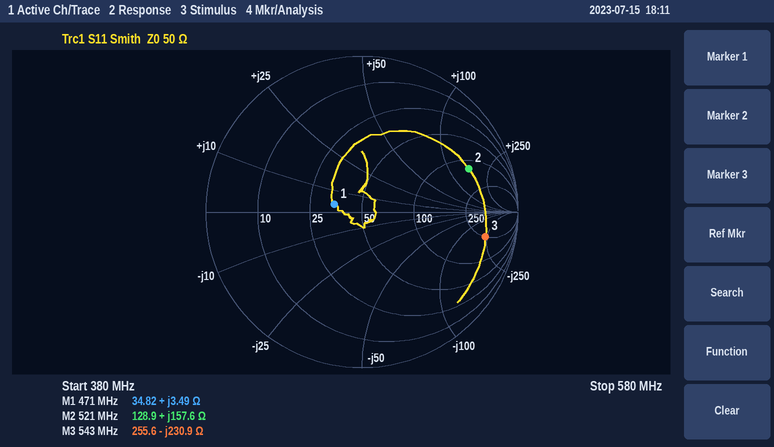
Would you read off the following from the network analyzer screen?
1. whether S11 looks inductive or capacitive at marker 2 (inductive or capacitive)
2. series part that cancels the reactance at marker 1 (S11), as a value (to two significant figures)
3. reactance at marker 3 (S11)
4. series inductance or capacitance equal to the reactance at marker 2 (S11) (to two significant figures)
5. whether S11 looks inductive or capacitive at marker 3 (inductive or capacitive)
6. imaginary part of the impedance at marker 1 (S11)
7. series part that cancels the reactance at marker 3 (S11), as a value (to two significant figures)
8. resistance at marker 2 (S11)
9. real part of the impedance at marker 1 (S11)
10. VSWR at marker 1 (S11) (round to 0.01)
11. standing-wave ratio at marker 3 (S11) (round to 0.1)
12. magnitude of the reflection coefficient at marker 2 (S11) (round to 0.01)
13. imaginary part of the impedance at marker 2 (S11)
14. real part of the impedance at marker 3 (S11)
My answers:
inductive
97 pF
-230.9 Ω
48 nH
capacitive
+3.49 Ω
68 nH
128.9 Ω
34.82 Ω
1.45
9.4
0.74
+157.6 Ω
255.6 Ω
